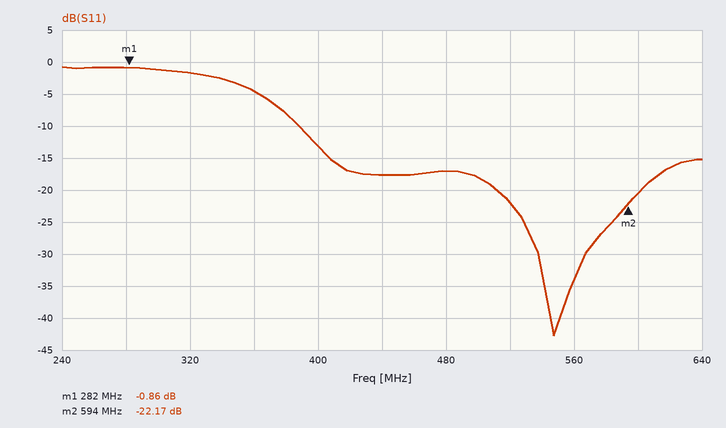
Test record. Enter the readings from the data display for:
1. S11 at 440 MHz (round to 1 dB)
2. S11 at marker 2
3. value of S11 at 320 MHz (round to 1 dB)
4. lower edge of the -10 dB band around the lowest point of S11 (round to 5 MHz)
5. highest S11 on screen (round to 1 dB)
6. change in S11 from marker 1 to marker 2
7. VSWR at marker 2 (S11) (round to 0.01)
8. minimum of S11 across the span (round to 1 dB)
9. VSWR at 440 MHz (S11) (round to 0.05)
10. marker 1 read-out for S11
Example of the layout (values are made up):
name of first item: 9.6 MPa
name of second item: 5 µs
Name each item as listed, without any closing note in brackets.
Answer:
S11 at 440 MHz: -18 dB
S11 at marker 2: -22.17 dB
value of S11 at 320 MHz: -2 dB
lower edge of the -10 dB band around the lowest point of S11: 390 MHz
highest S11 on screen: -1 dB
change in S11 from marker 1 to marker 2: -21.31 dB
VSWR at marker 2 (S11): 1.17
minimum of S11 across the span: -43 dB
VSWR at 440 MHz (S11): 1.30
marker 1 read-out for S11: -0.86 dB
